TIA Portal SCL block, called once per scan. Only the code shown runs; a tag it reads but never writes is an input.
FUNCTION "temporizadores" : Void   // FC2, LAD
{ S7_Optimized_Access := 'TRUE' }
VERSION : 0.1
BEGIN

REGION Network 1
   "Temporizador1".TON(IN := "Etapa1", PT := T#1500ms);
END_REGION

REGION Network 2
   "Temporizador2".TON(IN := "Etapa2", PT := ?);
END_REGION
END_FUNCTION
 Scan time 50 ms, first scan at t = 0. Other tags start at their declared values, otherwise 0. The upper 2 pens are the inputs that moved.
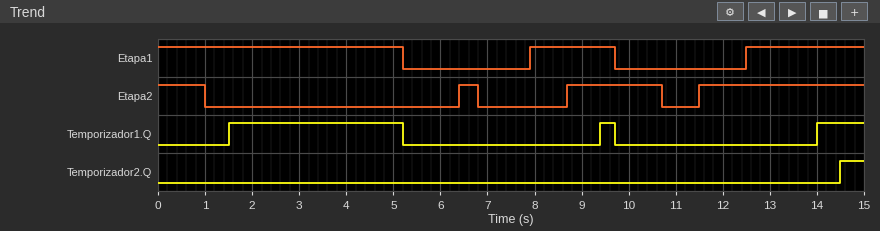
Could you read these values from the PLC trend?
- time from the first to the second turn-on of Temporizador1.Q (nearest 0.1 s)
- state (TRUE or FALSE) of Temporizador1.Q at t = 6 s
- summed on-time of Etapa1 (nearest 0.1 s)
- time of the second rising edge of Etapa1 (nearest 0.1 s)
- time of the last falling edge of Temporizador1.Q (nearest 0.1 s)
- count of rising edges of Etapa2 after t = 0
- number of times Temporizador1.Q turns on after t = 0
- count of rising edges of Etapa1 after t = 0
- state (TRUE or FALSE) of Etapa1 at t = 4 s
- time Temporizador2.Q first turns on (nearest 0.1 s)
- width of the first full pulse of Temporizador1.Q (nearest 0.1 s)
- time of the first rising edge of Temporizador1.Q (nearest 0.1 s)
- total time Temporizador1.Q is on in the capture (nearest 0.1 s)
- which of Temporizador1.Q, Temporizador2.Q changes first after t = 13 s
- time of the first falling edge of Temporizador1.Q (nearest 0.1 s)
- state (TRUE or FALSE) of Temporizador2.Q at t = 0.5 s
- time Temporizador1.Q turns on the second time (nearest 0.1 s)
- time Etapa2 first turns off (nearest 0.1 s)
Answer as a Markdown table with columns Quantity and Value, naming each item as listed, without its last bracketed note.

| Quantity | Value |
|---|---|
| time from the first to the second turn-on of Temporizador1.Q | 7.9 s |
| state (TRUE or FALSE) of Temporizador1.Q at t = 6 s | FALSE |
| summed on-time of Etapa1 | 9.5 s |
| time of the second rising edge of Etapa1 | 12.5 s |
| time of the last falling edge of Temporizador1.Q | 9.7 s |
| count of rising edges of Etapa2 after t = 0 | 3 |
| number of times Temporizador1.Q turns on after t = 0 | 3 |
| count of rising edges of Etapa1 after t = 0 | 2 |
| state (TRUE or FALSE) of Etapa1 at t = 4 s | TRUE |
| time Temporizador2.Q first turns on | 14.5 s |
| width of the first full pulse of Temporizador1.Q | 3.7 s |
| time of the first rising edge of Temporizador1.Q | 1.5 s |
| total time Temporizador1.Q is on in the capture | 5.0 s |
| which of Temporizador1.Q, Temporizador2.Q changes first after t = 13 s | Temporizador1.Q |
| time of the first falling edge of Temporizador1.Q | 5.2 s |
| state (TRUE or FALSE) of Temporizador2.Q at t = 0.5 s | FALSE |
| time Temporizador1.Q turns on the second time | 9.4 s |
| time Etapa2 first turns off | 1.0 s |
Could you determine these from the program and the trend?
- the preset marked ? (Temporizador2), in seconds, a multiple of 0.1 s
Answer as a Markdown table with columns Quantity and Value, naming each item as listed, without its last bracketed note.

| Quantity | Value |
|---|---|
| the preset marked ? (Temporizador2), in seconds, a multiple of 0.1 s | 3.0 s |
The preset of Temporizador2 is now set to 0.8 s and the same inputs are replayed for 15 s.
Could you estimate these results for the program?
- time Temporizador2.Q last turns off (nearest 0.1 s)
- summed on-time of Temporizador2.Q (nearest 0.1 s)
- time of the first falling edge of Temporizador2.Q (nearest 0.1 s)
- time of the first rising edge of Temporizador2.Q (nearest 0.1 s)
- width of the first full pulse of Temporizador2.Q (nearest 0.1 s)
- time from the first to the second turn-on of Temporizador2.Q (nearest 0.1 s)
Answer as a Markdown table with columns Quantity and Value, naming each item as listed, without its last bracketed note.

| Quantity | Value |
|---|---|
| time Temporizador2.Q last turns off | 10.7 s |
| summed on-time of Temporizador2.Q | 4.1 s |
| time of the first falling edge of Temporizador2.Q | 1.0 s |
| time of the first rising edge of Temporizador2.Q | 0.8 s |
| width of the first full pulse of Temporizador2.Q | 0.2 s |
| time from the first to the second turn-on of Temporizador2.Q | 8.7 s |
